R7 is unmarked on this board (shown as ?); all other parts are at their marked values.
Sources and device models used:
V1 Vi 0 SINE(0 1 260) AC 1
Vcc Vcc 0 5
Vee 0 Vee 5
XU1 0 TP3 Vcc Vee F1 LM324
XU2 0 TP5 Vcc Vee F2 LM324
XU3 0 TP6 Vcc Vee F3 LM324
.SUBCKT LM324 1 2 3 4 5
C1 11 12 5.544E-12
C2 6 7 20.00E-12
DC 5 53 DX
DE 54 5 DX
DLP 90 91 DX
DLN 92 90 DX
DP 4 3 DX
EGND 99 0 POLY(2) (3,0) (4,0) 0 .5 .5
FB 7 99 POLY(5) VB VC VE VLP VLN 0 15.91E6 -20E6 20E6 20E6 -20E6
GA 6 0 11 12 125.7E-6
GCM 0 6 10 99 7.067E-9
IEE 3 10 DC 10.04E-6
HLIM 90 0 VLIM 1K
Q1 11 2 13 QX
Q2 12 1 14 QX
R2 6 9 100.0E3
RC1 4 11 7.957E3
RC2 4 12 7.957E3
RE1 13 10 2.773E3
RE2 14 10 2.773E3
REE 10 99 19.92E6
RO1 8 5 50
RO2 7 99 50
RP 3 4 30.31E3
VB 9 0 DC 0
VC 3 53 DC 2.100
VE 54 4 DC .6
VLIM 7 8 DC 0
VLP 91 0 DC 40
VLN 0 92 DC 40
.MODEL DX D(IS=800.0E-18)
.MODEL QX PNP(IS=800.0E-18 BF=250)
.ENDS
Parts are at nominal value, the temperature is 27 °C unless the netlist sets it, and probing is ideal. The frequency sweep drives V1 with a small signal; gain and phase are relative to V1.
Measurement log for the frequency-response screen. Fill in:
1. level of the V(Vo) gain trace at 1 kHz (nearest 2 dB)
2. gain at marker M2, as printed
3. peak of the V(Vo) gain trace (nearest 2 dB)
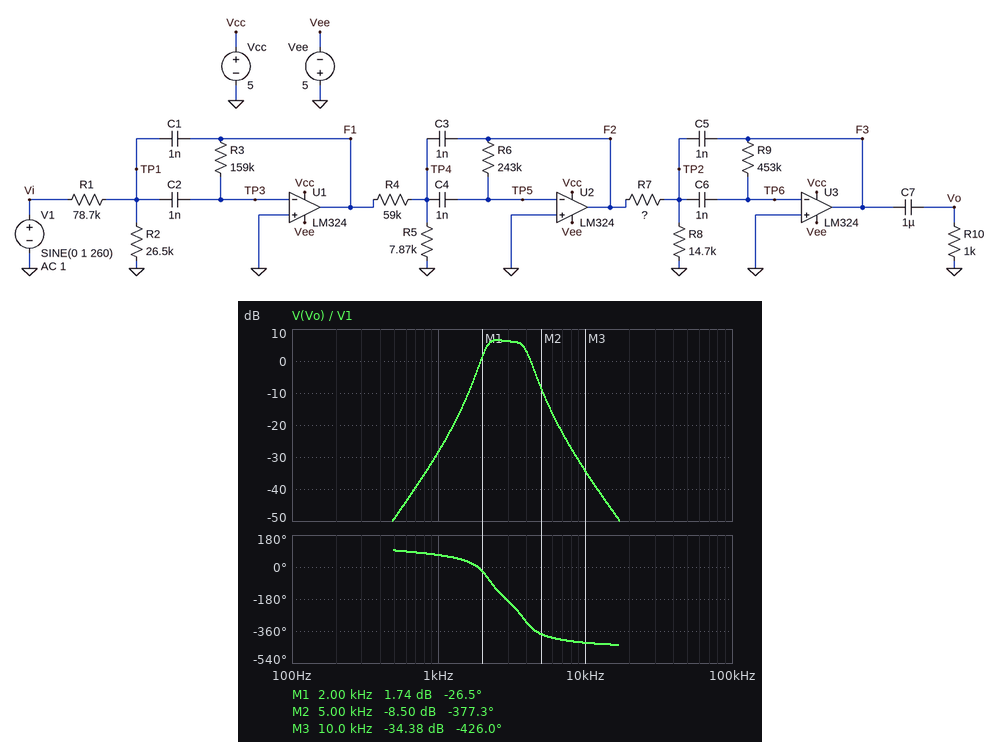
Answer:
-28 dB
-8.50 dB
6 dB
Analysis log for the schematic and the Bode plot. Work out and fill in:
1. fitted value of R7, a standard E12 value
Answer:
56 kΩ
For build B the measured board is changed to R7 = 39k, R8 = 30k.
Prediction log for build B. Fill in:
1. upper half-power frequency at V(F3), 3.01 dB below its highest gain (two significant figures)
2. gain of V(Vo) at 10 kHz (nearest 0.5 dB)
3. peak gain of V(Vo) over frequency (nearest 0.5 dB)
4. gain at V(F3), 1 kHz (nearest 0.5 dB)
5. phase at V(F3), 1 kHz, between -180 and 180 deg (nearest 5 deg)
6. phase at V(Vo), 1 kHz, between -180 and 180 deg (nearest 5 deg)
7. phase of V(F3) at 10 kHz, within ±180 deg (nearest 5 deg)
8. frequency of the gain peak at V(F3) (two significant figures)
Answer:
4.0 kHz
-31.5 dB
7.5 dB
-21.0 dB
50 deg
60 deg
-65 deg
3.4 kHz
